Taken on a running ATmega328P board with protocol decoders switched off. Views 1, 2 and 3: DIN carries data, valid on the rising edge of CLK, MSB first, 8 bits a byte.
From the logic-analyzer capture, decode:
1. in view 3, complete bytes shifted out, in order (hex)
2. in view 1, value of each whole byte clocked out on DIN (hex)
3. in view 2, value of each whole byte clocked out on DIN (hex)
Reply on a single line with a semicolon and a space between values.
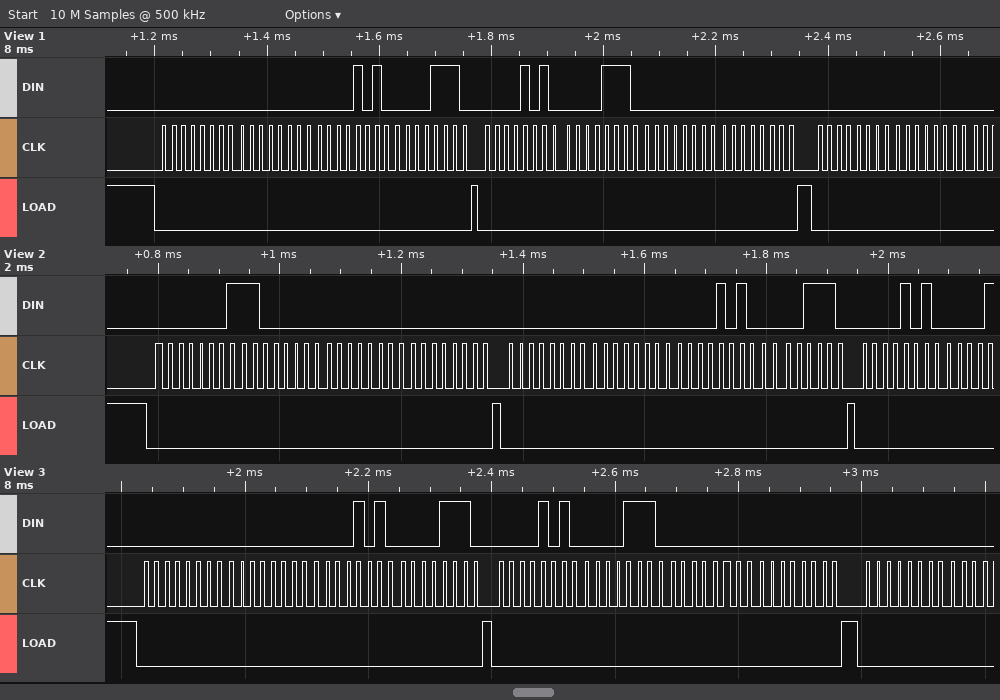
0x00 0x00 0x0A 0x0E 0x0A 0x0E 0x00 0x00 0x00; 00 00 0A 0E 0A 0E 00 00 00 00; 01 C0 00 00 00 00 0A 0E 0A
